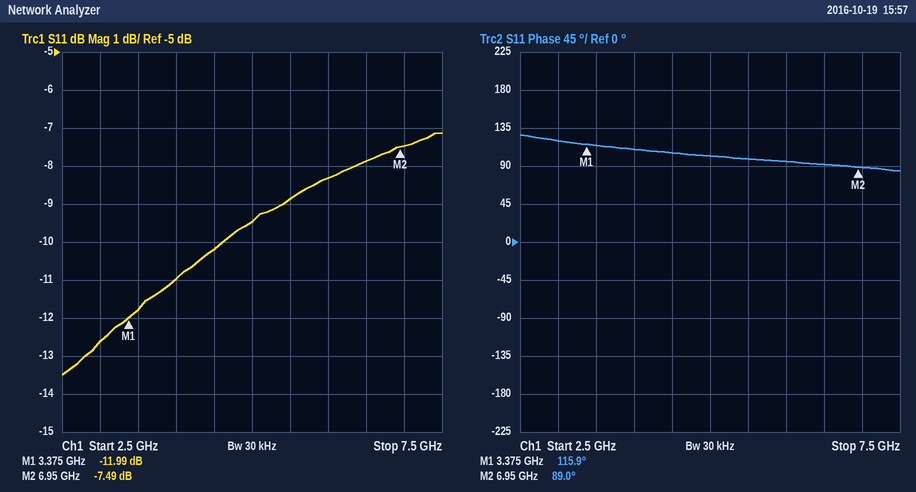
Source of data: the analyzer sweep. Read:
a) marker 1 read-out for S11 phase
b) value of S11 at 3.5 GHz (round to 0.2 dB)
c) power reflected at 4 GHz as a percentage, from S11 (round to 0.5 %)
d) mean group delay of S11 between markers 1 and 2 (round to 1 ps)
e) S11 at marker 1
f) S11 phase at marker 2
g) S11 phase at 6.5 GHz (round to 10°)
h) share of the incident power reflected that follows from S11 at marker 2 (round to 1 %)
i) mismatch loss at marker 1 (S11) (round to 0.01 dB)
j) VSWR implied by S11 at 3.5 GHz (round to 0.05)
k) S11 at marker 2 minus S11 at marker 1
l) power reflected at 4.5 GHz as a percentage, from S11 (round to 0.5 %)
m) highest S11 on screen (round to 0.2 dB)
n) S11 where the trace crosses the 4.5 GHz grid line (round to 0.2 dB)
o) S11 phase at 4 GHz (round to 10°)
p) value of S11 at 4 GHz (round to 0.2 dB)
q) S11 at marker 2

115.9°
-11.8 dB
8.0 %
21 ps
-11.99 dB
89.0°
90°
18 %
0.28 dB
1.70
4.50 dB
9.5 %
-7.2 dB
-10.2 dB
110°
-11.0 dB
-7.49 dB
